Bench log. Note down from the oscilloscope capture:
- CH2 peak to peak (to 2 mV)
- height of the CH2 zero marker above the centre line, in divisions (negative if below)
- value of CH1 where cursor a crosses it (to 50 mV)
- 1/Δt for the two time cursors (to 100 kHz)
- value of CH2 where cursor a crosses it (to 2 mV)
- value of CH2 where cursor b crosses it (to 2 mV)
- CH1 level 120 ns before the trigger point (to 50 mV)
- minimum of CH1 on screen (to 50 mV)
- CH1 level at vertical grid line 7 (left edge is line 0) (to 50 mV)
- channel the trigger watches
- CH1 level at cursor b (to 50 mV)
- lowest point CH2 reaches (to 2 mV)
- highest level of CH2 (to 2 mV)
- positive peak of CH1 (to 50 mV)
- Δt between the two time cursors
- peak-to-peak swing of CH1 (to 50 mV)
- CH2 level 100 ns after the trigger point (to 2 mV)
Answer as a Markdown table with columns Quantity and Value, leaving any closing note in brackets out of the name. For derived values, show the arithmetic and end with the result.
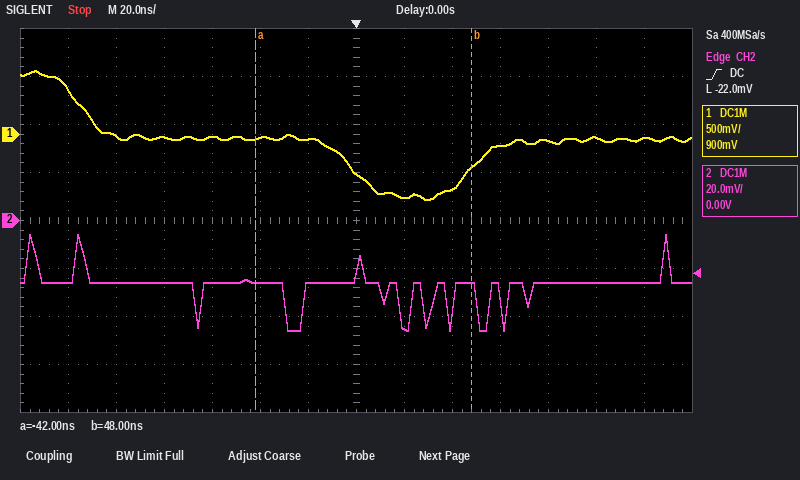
| Quantity | Value |
|---|---|
| CH2 peak to peak | -6 mV − (-46 mV) = 40 mV |
| height of the CH2 zero marker above the centre line, in divisions | 0.0 div |
| value of CH1 where cursor a crosses it | -50 mV |
| 1/Δt for the two time cursors | 1 / 90 ns ≈ 11.1 MHz |
| value of CH2 where cursor a crosses it | -26 mV |
| value of CH2 where cursor b crosses it | -28 mV |
| CH1 level 120 ns before the trigger point | 450 mV |
| minimum of CH1 on screen | -700 mV |
| CH1 level at vertical grid line 7 (left edge is line 0) | -400 mV |
| channel the trigger watches | CH2 |
| CH1 level at cursor b | -350 mV |
| lowest point CH2 reaches | -46 mV |
| highest level of CH2 | -6 mV |
| positive peak of CH1 | 650 mV |
| Δt between the two time cursors | 48 ns − (-42 ns) = 90 ns |
| peak-to-peak swing of CH1 | 650 mV − (-700 mV) = 1.35 V |
| CH2 level 100 ns after the trigger point | -26 mV |
